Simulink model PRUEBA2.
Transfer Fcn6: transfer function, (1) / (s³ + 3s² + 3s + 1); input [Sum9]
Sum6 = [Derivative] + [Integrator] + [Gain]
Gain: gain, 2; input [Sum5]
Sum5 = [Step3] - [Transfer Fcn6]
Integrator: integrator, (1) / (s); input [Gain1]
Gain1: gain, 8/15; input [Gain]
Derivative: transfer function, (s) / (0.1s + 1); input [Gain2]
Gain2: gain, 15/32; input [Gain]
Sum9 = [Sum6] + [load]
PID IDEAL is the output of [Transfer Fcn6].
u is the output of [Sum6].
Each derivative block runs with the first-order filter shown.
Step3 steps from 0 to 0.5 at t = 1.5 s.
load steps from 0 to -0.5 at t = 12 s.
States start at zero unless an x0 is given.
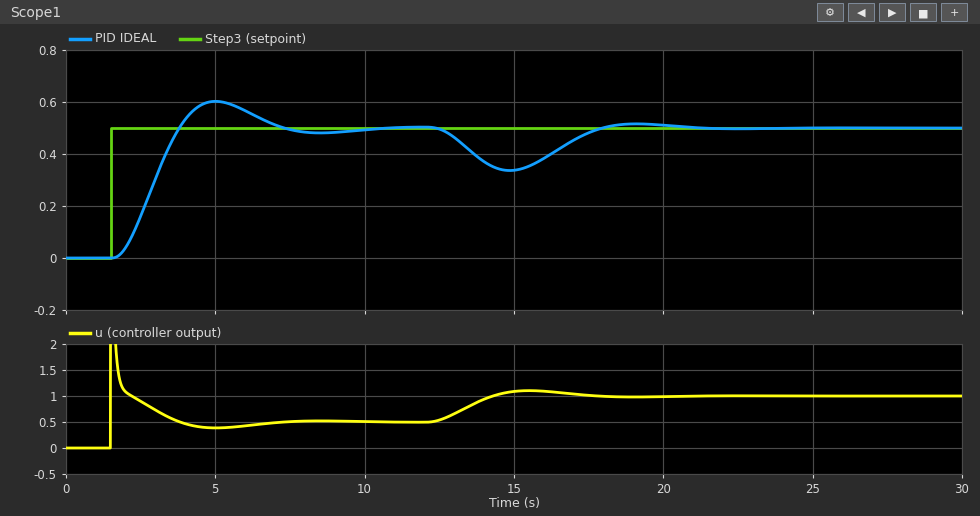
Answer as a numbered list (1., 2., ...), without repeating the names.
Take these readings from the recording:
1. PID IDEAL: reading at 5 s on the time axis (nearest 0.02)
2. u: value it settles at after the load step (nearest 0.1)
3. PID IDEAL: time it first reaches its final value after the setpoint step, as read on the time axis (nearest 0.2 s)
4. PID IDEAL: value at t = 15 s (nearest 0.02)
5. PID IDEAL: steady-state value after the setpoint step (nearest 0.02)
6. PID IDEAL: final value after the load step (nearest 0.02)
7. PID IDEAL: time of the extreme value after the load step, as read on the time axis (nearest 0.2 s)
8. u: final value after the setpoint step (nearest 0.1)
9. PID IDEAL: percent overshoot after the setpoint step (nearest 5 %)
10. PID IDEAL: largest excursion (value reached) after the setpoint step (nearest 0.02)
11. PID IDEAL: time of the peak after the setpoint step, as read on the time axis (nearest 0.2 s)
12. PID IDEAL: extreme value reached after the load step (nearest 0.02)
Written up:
1. 0.60
2. 1.0
3. 3.8 s
4. 0.34
5. 0.50
6. 0.50
7. 14.8 s
8. 0.5
9. 20 %
10. 0.60
11. 5.0 s
12. 0.34
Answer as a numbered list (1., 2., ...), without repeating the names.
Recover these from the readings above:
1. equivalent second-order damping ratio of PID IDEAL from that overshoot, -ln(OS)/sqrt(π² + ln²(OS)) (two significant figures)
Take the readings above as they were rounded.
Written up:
1. 0.46
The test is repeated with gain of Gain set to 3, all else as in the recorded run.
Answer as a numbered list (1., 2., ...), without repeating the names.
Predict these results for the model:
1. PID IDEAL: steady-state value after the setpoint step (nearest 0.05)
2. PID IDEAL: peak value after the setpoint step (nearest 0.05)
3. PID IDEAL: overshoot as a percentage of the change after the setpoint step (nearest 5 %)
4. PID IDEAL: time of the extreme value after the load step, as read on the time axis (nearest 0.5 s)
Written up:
1. 0.50
2. 0.65
3. 30 %
4. 14.5 s
